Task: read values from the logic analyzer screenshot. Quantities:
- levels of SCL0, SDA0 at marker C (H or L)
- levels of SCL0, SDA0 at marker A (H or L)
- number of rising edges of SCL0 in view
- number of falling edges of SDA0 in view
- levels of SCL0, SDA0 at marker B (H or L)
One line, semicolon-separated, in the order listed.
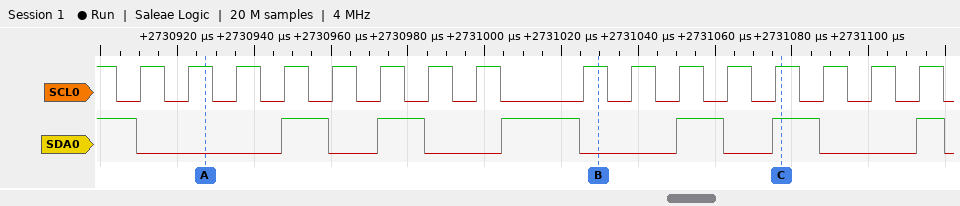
SCL0=H, SDA0=H; SCL0=H, SDA0=L; 16; 7; SCL0=H, SDA0=L
